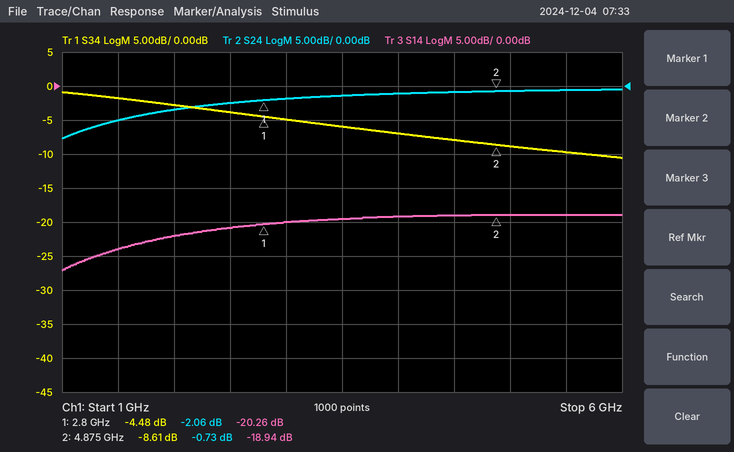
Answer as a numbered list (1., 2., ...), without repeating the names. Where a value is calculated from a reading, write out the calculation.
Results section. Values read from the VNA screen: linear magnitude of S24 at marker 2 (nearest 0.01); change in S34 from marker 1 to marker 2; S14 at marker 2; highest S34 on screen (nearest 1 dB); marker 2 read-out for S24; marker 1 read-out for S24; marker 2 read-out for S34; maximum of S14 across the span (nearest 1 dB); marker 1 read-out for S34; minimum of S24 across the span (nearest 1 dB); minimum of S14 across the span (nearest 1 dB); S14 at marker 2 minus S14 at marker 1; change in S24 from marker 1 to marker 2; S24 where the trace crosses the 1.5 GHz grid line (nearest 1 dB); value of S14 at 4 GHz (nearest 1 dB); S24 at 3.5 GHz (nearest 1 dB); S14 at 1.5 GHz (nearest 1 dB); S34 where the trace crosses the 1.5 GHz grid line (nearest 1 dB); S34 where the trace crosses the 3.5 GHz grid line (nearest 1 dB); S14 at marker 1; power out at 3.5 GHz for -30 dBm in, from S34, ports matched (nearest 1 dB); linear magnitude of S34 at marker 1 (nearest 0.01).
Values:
1. 10^(-0.73/20) ≈ 0.92
2. -8.61 − (-4.48) = -4.13 dB
3. -18.94 dB
4. -1 dB
5. -0.73 dB
6. -2.06 dB
7. -8.61 dB
8. -19 dB
9. -4.48 dB
10. -8 dB
11. -27 dB
12. -18.94 − (-20.26) = 1.32 dB
13. -0.73 − (-2.06) = 1.33 dB
14. -5 dB
15. -19 dB
16. -1 dB
17. -24 dB
18. -2 dB
19. -6 dB
20. -20.26 dB
21. -30 dBm + (-6 dB) = -36 dBm
22. 10^(-4.48/20) ≈ 0.60
